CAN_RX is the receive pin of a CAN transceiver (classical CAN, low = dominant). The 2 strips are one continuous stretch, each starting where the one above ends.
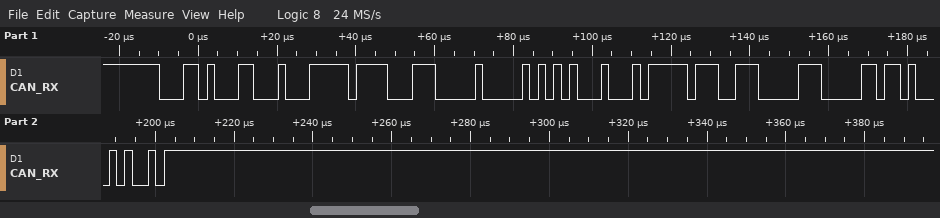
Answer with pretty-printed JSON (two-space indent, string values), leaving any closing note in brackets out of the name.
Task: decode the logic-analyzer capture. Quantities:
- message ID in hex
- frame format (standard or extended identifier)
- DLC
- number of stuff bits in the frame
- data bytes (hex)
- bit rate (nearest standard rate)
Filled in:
{
  "message ID in hex": "0x1A3",
  "frame format": "standard",
  "DLC": "8",
  "number of stuff bits in the frame": "6",
  "data bytes": "FF 8E 00 2A 22 FF 38 30",
  "bit rate": "500 kbit/s"
}
